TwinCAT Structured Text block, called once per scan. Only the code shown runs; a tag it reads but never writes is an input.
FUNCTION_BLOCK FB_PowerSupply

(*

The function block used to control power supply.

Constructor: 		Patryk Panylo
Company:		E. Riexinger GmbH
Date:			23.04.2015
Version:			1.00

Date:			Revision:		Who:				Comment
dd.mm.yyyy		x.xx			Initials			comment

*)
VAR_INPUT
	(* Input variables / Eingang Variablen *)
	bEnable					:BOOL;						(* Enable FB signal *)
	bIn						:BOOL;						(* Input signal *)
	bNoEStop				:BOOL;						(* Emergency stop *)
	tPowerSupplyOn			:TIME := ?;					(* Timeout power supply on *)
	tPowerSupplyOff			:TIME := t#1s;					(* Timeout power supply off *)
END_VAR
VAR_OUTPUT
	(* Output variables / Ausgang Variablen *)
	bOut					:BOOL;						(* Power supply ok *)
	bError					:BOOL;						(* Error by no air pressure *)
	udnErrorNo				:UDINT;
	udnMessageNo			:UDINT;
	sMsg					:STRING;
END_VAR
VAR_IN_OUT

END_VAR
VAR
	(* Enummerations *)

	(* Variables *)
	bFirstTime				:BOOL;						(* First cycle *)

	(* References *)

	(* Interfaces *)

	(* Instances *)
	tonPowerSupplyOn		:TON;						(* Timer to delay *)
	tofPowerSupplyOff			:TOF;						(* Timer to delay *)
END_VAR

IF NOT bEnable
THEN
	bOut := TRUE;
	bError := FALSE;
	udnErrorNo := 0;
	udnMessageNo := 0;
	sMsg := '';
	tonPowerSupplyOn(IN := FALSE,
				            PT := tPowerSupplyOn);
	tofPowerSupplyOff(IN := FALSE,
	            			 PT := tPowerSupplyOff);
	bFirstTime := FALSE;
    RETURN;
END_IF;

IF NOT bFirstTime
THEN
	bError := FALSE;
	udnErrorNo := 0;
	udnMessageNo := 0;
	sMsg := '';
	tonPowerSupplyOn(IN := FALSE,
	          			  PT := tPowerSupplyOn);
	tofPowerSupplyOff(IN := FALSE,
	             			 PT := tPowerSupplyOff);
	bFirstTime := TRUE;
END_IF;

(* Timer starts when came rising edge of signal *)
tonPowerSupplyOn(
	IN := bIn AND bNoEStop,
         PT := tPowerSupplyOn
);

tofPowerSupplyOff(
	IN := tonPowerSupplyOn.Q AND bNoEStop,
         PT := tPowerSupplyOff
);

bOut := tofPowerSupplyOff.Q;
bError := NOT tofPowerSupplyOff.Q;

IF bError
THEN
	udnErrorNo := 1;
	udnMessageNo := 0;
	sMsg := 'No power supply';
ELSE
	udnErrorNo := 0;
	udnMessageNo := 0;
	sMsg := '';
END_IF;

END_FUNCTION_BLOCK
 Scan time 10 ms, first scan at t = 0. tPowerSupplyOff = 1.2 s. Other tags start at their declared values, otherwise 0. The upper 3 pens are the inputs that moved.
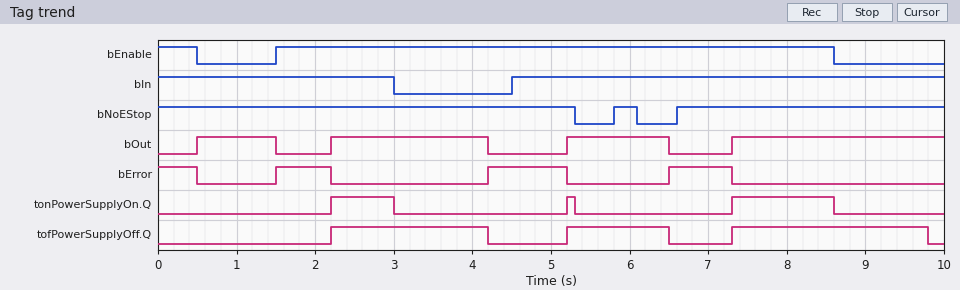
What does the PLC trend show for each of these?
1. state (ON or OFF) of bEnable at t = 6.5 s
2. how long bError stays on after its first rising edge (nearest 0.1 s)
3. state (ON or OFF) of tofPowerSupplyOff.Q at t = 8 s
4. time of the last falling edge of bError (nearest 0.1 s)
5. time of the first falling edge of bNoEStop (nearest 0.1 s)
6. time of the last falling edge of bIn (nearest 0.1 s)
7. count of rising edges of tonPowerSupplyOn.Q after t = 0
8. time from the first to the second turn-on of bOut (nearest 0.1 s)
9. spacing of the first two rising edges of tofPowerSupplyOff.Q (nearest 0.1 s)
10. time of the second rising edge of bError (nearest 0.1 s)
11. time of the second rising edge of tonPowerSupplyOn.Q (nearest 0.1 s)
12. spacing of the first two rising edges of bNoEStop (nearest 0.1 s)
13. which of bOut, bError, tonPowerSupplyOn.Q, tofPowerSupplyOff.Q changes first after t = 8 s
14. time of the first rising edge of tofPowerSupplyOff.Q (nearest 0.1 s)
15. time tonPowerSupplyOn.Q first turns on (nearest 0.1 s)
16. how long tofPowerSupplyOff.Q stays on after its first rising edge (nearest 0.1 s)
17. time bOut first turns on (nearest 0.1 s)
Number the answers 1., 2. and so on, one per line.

1. ON
2. 0.7 s
3. ON
4. 7.3 s
5. 5.3 s
6. 3.0 s
7. 3
8. 1.7 s
9. 3.0 s
10. 4.2 s
11. 5.2 s
12. 0.8 s
13. tonPowerSupplyOn.Q
14. 2.2 s
15. 2.2 s
16. 2.0 s
17. 0.5 s
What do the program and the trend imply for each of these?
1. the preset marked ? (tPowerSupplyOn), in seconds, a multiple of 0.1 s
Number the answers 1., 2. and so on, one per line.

1. 0.7 s
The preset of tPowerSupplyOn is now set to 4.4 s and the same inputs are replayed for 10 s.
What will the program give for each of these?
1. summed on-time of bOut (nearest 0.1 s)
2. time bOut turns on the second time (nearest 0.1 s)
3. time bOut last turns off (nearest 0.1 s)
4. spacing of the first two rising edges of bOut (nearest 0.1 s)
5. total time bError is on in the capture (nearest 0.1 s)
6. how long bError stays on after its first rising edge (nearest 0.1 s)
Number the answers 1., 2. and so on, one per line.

1. 2.4 s
2. 8.6 s
3. 1.5 s
4. 8.1 s
5. 7.6 s
6. 7.1 s
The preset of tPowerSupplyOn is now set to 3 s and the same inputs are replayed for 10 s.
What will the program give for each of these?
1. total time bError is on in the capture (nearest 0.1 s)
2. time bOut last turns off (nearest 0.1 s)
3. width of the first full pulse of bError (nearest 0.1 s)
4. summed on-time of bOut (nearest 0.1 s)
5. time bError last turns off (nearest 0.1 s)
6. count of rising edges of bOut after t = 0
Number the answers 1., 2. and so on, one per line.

1. 7.6 s
2. 1.5 s
3. 7.1 s
4. 2.4 s
5. 8.6 s
6. 2
